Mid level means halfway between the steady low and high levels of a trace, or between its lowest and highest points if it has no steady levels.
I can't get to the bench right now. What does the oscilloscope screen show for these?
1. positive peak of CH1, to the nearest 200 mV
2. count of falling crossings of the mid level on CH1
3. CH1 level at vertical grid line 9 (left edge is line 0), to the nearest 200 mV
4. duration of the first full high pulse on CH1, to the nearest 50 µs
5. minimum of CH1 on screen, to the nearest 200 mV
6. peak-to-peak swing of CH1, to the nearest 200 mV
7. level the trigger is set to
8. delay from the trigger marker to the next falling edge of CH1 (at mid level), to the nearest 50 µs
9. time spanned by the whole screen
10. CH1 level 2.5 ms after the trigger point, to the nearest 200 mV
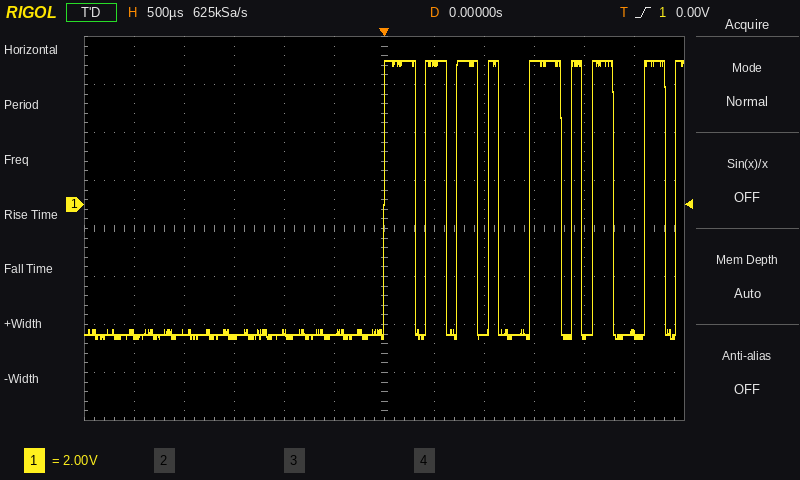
6.0 V
8
6.0 V
300 µs
-5.6 V
11.6 V
0.00 V
300 µs
6 ms
-5.4 V
